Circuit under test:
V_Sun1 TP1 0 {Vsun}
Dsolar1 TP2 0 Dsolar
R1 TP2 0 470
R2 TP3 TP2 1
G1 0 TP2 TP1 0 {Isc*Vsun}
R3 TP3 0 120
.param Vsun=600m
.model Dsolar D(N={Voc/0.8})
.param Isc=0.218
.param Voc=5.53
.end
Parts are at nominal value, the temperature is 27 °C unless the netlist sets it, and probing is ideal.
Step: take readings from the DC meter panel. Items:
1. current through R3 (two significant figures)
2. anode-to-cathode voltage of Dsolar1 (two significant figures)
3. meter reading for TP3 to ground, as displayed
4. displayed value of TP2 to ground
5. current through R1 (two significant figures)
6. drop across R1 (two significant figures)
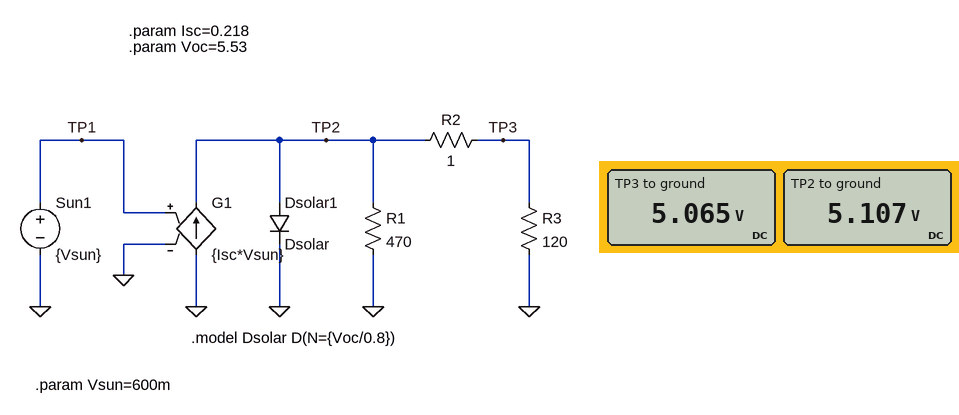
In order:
42 mA
5.1 V
5.065 V
5.107 V
11 mA
5.1 V
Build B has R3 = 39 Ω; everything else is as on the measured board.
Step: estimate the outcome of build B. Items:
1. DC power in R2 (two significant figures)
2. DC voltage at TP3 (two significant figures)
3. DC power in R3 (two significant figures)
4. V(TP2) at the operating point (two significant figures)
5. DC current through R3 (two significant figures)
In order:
5.2 mW
2.8 V
200 mW
2.9 V
72 mA
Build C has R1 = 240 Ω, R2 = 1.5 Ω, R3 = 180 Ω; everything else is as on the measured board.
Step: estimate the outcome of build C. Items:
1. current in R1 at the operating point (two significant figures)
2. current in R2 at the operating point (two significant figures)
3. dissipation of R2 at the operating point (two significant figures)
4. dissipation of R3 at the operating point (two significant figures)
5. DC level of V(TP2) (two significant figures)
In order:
21 mA
28 mA
1.2 mW
140 mW
5.1 V
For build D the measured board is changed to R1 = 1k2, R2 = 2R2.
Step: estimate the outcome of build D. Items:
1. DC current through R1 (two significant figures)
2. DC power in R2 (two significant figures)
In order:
4.3 mA
3.9 mW
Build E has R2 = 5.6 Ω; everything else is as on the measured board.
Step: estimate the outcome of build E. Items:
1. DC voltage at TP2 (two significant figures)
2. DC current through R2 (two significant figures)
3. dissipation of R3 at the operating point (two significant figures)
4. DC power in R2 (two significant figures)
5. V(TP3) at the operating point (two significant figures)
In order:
5.1 V
41 mA
200 mW
9.3 mW
4.9 V
